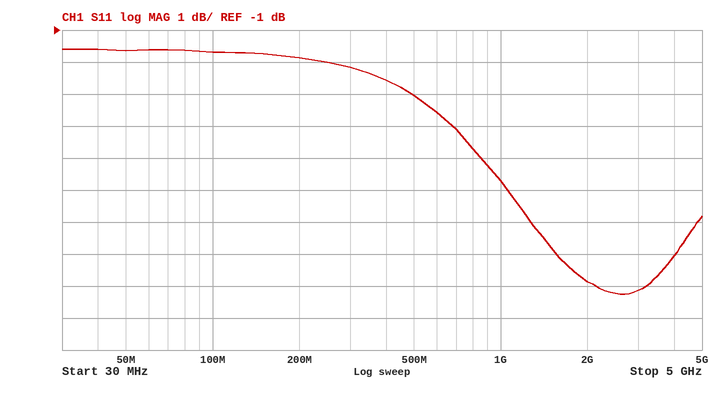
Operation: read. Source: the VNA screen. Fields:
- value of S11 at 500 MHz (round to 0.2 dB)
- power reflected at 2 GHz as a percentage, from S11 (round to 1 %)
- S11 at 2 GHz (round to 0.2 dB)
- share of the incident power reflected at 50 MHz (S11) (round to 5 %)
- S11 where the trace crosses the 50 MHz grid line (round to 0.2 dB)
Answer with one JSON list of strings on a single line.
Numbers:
["-3.0 dB", "13 %", "-8.8 dB", "70 %", "-1.6 dB"]
